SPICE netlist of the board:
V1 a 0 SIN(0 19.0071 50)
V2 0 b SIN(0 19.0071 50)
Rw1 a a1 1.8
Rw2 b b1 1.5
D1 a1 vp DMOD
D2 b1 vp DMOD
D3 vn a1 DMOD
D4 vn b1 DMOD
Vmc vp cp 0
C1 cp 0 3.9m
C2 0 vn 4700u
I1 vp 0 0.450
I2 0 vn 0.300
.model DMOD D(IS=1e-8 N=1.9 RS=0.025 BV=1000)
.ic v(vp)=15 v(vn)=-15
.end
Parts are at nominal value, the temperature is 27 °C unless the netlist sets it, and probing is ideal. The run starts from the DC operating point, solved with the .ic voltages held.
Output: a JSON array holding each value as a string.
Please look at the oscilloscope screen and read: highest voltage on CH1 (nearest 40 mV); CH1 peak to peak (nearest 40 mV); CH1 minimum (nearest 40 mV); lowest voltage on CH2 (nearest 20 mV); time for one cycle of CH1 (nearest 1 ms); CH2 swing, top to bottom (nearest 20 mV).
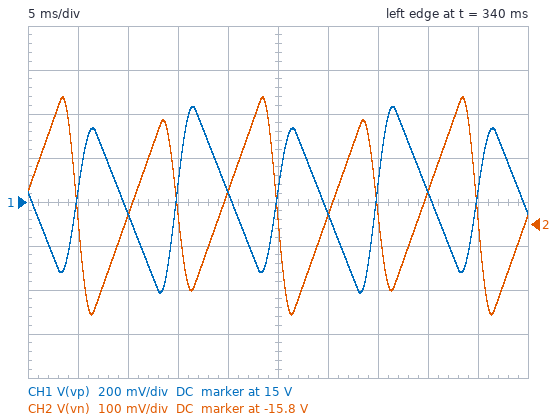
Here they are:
["15.44 V", "840 mV", "14.60 V", "-16.00 V", "10 ms", "500 mV"]
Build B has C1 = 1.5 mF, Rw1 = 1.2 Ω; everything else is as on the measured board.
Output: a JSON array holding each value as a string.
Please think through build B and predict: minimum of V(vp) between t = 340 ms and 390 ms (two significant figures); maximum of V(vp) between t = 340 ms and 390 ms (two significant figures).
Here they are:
["14 V", "16 V"]
